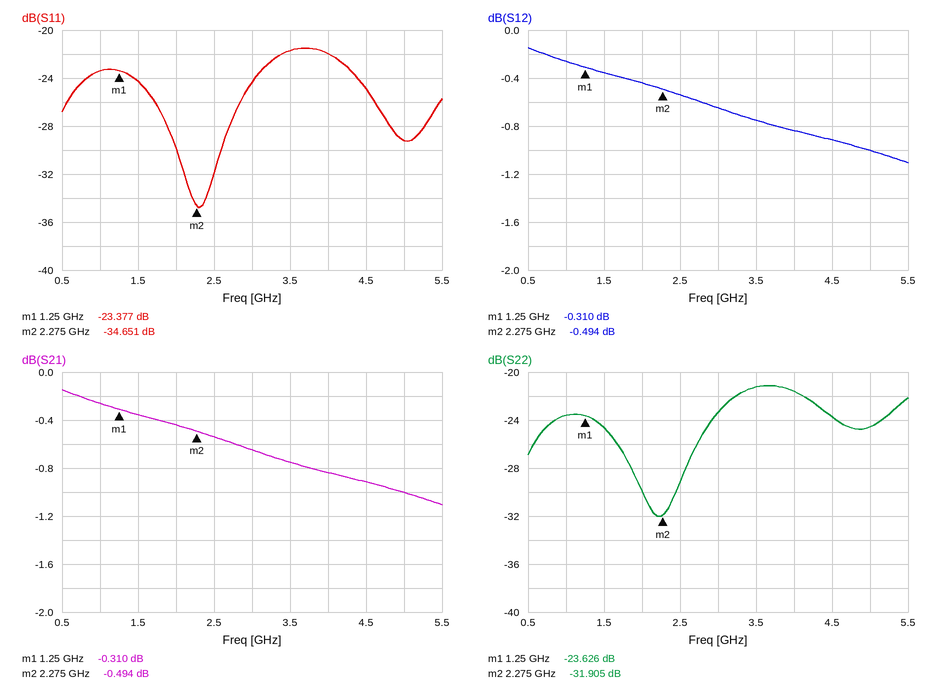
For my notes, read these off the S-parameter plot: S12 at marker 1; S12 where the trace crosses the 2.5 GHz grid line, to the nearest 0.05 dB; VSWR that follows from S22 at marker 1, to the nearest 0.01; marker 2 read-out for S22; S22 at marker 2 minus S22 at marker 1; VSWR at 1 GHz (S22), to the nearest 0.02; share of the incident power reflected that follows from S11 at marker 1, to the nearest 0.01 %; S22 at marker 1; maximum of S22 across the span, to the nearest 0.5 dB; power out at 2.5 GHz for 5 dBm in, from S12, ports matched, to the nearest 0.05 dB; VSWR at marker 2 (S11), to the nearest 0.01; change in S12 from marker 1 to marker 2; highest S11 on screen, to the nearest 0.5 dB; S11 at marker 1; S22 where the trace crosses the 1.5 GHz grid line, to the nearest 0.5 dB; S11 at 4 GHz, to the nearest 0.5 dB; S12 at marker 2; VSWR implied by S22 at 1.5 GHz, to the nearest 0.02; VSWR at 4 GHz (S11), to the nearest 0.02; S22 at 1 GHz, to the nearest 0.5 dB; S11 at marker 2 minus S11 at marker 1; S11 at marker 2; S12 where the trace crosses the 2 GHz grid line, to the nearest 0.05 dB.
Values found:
-0.310 dB
-0.55 dB
1.14
-31.905 dB
-8.279 dB
1.14
0.46 %
-23.626 dB
-21.0 dB
4.45 dBm
1.04
-0.184 dB
-21.5 dB
-23.377 dB
-24.5 dB
-22.0 dB
-0.494 dB
1.12
1.18
-23.5 dB
-11.274 dB
-34.651 dB
-0.45 dB
